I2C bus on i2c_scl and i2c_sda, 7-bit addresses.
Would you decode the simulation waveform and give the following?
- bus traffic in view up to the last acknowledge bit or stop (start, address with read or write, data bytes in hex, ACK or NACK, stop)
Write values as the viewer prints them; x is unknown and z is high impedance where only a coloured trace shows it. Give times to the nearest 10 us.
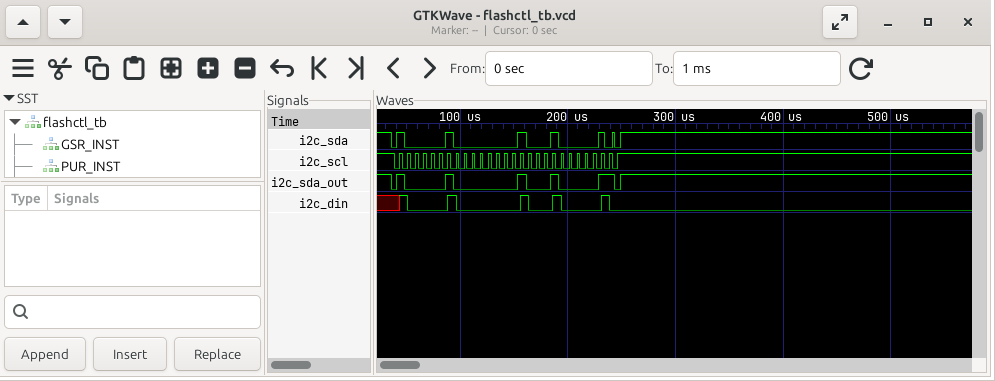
start, address 41 write ACK, 02 ACK, 41 ACK, stop
